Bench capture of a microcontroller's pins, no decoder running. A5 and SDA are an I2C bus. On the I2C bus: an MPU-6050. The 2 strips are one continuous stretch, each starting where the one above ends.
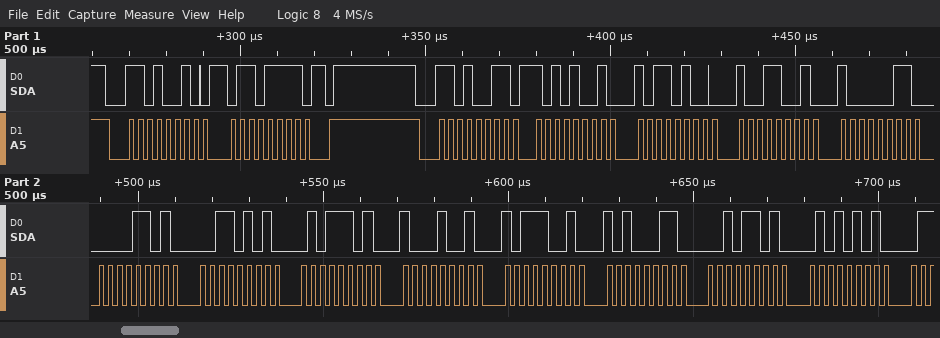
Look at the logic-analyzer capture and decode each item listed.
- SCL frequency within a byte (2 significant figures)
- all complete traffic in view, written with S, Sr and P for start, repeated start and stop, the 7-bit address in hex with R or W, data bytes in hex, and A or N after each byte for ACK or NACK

400 kHz
S 69W A 6F A P S 69R A A9 A B4 A 99 A 83 A 0D A 35 A 5D A 89 A B9 A A3 A 2D A 55 A
